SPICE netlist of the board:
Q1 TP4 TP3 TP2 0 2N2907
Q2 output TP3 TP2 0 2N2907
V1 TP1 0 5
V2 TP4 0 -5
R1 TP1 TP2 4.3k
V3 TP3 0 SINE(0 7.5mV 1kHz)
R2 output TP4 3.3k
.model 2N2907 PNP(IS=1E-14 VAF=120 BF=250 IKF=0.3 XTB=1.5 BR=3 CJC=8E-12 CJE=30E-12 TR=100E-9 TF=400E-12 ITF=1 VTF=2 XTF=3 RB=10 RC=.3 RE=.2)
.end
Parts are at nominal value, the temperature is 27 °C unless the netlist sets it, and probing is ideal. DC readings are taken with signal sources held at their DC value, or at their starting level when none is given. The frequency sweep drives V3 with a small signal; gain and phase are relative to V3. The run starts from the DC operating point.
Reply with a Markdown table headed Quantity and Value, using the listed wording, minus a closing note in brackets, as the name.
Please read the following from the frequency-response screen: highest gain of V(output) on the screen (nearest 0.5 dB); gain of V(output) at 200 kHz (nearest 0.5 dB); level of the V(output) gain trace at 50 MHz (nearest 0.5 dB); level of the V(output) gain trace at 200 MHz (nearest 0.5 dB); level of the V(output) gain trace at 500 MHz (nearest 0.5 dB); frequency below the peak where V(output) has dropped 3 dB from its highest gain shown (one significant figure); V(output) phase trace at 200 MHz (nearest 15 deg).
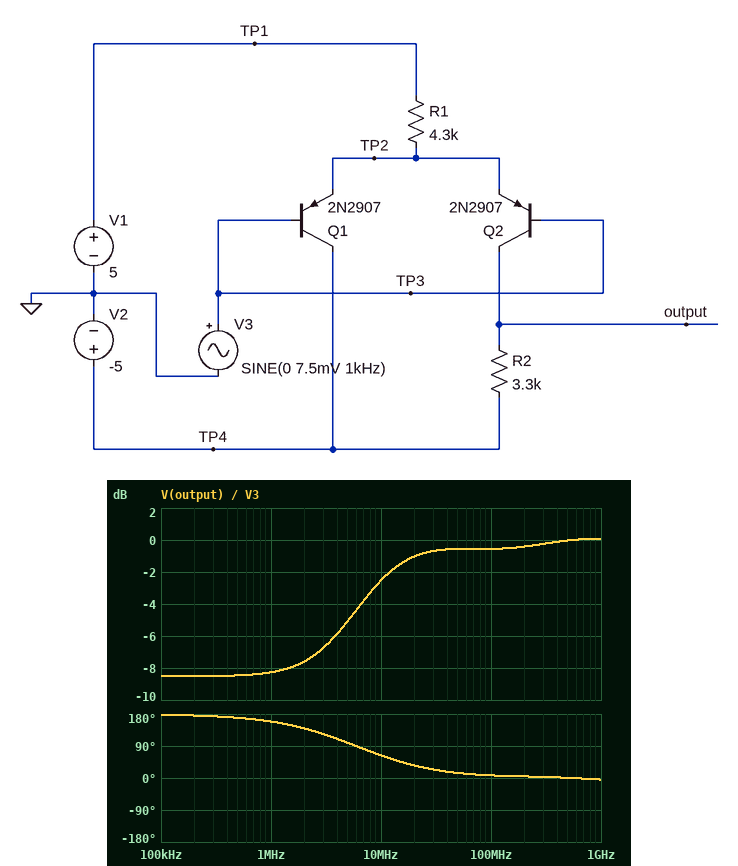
| Quantity | Value |
|---|---|
| highest gain of V(output) on the screen | 0 dB |
| gain of V(output) at 200 kHz | -8.5 dB |
| level of the V(output) gain trace at 50 MHz | -0.5 dB |
| level of the V(output) gain trace at 200 MHz | -0.5 dB |
| level of the V(output) gain trace at 500 MHz | 0 dB |
| frequency below the peak where V(output) has dropped 3 dB from its highest gain shown | 9 MHz |
| V(output) phase trace at 200 MHz | 0 deg |
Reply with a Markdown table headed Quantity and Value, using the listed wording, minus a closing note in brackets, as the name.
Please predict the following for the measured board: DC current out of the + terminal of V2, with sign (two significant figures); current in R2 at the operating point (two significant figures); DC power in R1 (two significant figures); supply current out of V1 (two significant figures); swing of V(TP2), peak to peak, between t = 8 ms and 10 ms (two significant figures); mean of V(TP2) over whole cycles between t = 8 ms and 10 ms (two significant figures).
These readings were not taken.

| Quantity | Value |
|---|---|
| DC current out of the + terminal of V2, with sign | -1.0 mA |
| current in R2 at the operating point | 500 µA |
| DC power in R1 | 4.4 mW |
| supply current out of V1 | 1.0 mA |
| swing of V(TP2), peak to peak, between t = 8 ms and 10 ms | 15 mV |
| mean of V(TP2) over whole cycles between t = 8 ms and 10 ms | 640 mV |
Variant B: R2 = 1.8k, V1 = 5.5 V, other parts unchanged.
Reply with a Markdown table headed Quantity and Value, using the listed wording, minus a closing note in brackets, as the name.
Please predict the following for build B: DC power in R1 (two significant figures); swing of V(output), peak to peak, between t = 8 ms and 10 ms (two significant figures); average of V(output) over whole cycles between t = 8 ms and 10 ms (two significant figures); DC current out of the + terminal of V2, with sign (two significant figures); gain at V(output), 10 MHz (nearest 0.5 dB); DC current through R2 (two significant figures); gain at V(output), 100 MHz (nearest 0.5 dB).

| Quantity | Value |
|---|---|
| DC power in R1 | 5.5 mW |
| swing of V(output), peak to peak, between t = 8 ms and 10 ms | 3.1 mV |
| average of V(output) over whole cycles between t = 8 ms and 10 ms | -4.0 V |
| DC current out of the + terminal of V2, with sign | -1.1 mA |
| gain at V(output), 10 MHz | -6.0 dB |
| DC current through R2 | 560 µA |
| gain at V(output), 100 MHz | -1.0 dB |
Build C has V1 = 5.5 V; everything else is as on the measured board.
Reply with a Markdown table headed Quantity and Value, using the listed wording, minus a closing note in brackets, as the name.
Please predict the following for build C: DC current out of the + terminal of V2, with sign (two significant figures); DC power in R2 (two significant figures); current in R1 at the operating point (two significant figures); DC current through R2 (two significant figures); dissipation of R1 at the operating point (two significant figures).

| Quantity | Value |
|---|---|
| DC current out of the + terminal of V2, with sign | -1.1 mA |
| DC power in R2 | 1.0 mW |
| current in R1 at the operating point | 1.1 mA |
| DC current through R2 | 560 µA |
| dissipation of R1 at the operating point | 5.5 mW |
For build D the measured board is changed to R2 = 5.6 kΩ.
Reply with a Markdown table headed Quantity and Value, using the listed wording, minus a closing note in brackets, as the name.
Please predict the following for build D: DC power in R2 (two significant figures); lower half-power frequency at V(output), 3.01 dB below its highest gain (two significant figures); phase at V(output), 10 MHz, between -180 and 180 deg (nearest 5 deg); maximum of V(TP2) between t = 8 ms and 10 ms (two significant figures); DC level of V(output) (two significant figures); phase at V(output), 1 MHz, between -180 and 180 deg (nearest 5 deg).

| Quantity | Value |
|---|---|
| DC power in R2 | 1.4 mW |
| lower half-power frequency at V(output), 3.01 dB below its highest gain | 2.6 MHz |
| phase at V(output), 10 MHz, between -180 and 180 deg | 45 deg |
| maximum of V(TP2) between t = 8 ms and 10 ms | 640 mV |
| DC level of V(output) | -2.2 V |
| phase at V(output), 1 MHz, between -180 and 180 deg | 150 deg |
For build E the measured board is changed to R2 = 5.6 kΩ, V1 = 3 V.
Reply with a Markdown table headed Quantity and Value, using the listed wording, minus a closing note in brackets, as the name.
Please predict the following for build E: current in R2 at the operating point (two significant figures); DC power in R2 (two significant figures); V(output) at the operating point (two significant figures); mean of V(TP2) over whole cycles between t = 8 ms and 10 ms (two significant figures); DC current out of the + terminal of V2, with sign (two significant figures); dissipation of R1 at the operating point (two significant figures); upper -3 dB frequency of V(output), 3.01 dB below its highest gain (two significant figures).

| Quantity | Value |
|---|---|
| current in R2 at the operating point | 270 µA |
| DC power in R2 | 420 µW |
| V(output) at the operating point | -3.5 V |
| mean of V(TP2) over whole cycles between t = 8 ms and 10 ms | 620 mV |
| DC current out of the + terminal of V2, with sign | -550 µA |
| dissipation of R1 at the operating point | 1.3 mW |
| upper -3 dB frequency of V(output), 3.01 dB below its highest gain | 7.8 GHz |
